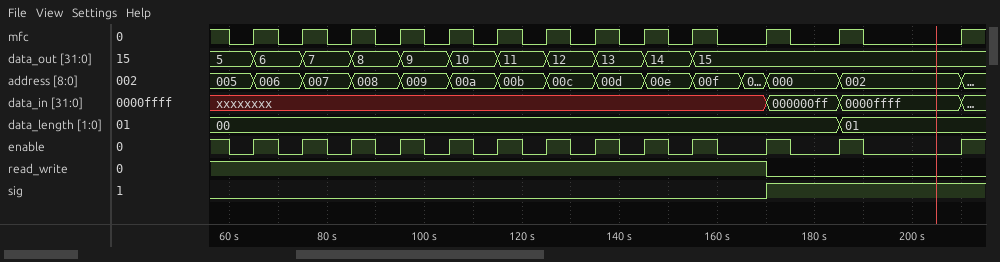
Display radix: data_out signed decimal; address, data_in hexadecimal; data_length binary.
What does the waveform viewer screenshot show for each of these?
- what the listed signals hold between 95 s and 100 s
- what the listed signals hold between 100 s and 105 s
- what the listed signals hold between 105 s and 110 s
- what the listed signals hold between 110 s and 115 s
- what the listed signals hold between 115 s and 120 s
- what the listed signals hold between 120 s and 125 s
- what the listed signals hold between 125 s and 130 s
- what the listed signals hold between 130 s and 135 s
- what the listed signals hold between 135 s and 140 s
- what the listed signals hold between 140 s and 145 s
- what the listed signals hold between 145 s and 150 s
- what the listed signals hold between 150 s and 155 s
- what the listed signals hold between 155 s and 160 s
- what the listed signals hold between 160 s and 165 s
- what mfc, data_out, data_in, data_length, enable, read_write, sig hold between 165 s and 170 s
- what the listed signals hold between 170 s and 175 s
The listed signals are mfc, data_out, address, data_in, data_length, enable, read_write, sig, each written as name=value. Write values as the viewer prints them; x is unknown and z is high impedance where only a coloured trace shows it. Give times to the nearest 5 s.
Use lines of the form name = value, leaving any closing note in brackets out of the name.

what the listed signals hold between 95 s and 100 s = mfc=1, data_out=9, address=009, data_in=xxxxxxxx, data_length=00, enable=1, read_write=1, sig=0
what the listed signals hold between 100 s and 105 s = mfc=0, data_out=9, address=009, data_in=xxxxxxxx, data_length=00, enable=0, read_write=1, sig=0
what the listed signals hold between 105 s and 110 s = mfc=1, data_out=10, address=00a, data_in=xxxxxxxx, data_length=00, enable=1, read_write=1, sig=0
what the listed signals hold between 110 s and 115 s = mfc=0, data_out=10, address=00a, data_in=xxxxxxxx, data_length=00, enable=0, read_write=1, sig=0
what the listed signals hold between 115 s and 120 s = mfc=1, data_out=11, address=00b, data_in=xxxxxxxx, data_length=00, enable=1, read_write=1, sig=0
what the listed signals hold between 120 s and 125 s = mfc=0, data_out=11, address=00b, data_in=xxxxxxxx, data_length=00, enable=0, read_write=1, sig=0
what the listed signals hold between 125 s and 130 s = mfc=1, data_out=12, address=00c, data_in=xxxxxxxx, data_length=00, enable=1, read_write=1, sig=0
what the listed signals hold between 130 s and 135 s = mfc=0, data_out=12, address=00c, data_in=xxxxxxxx, data_length=00, enable=0, read_write=1, sig=0
what the listed signals hold between 135 s and 140 s = mfc=1, data_out=13, address=00d, data_in=xxxxxxxx, data_length=00, enable=1, read_write=1, sig=0
what the listed signals hold between 140 s and 145 s = mfc=0, data_out=13, address=00d, data_in=xxxxxxxx, data_length=00, enable=0, read_write=1, sig=0
what the listed signals hold between 145 s and 150 s = mfc=1, data_out=14, address=00e, data_in=xxxxxxxx, data_length=00, enable=1, read_write=1, sig=0
what the listed signals hold between 150 s and 155 s = mfc=0, data_out=14, address=00e, data_in=xxxxxxxx, data_length=00, enable=0, read_write=1, sig=0
what the listed signals hold between 155 s and 160 s = mfc=1, data_out=15, address=00f, data_in=xxxxxxxx, data_length=00, enable=1, read_write=1, sig=0
what the listed signals hold between 160 s and 165 s = mfc=0, data_out=15, address=00f, data_in=xxxxxxxx, data_length=00, enable=0, read_write=1, sig=0
what mfc, data_out, data_in, data_length, enable, read_write, sig hold between 165 s and 170 s = mfc=0, data_out=15, data_in=xxxxxxxx, data_length=00, enable=0, read_write=1, sig=0
what the listed signals hold between 170 s and 175 s = mfc=1, data_out=15, address=000, data_in=000000ff, data_length=00, enable=1, read_write=0, sig=1
